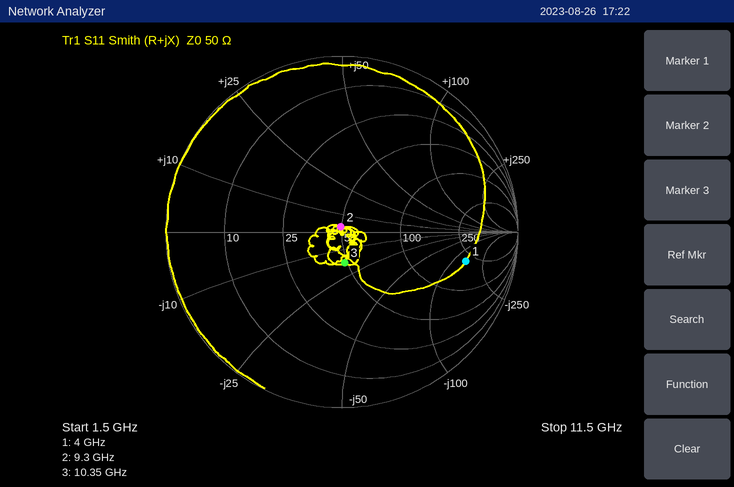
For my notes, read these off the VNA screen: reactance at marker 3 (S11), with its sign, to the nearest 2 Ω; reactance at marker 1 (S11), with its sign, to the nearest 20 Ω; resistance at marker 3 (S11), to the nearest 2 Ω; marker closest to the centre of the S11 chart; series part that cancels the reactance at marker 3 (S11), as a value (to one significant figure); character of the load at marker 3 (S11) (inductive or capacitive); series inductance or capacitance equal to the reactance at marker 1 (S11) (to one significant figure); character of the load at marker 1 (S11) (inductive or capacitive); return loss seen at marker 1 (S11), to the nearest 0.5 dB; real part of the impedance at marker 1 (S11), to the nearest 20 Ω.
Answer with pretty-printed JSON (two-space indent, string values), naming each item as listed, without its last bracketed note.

{
  "reactance at marker 3 (S11), with its sign, to the nearest 2 Ω": "-18 Ω",
  "reactance at marker 1 (S11), with its sign, to the nearest 20 Ω": "-140 Ω",
  "resistance at marker 3 (S11), to the nearest 2 Ω": "48 Ω",
  "marker closest to the centre of the S11 chart": "marker 2",
  "series part that cancels the reactance at marker 3 (S11), as a value": "300 pH",
  "character of the load at marker 3 (S11)": "capacitive",
  "series inductance or capacitance equal to the reactance at marker 1 (S11)": "300 fF",
  "character of the load at marker 1 (S11)": "capacitive",
  "return loss seen at marker 1 (S11), to the nearest 0.5 dB": "3.0 dB",
  "real part of the impedance at marker 1 (S11), to the nearest 20 Ω": "200 Ω"
}
